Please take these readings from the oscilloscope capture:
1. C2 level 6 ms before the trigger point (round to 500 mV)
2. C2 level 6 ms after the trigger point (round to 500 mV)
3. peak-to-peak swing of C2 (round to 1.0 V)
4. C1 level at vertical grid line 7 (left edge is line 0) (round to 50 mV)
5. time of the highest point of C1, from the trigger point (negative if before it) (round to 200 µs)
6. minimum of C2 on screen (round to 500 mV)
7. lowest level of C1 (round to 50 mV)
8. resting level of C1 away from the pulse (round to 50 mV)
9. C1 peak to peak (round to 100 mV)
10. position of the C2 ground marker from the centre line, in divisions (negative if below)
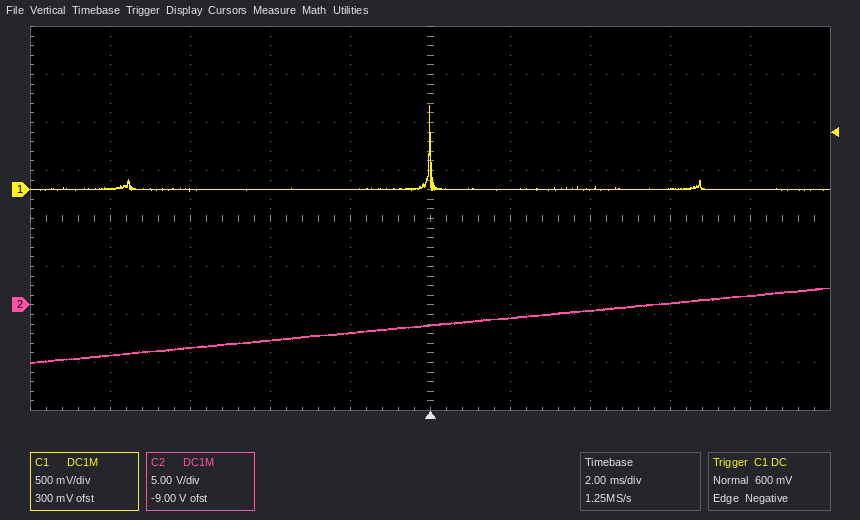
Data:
-4.5 V
0.0 V
8.0 V
0 mV
0.0 ms
-6.0 V
0 mV
0 mV
900 mV
-1.8 div
